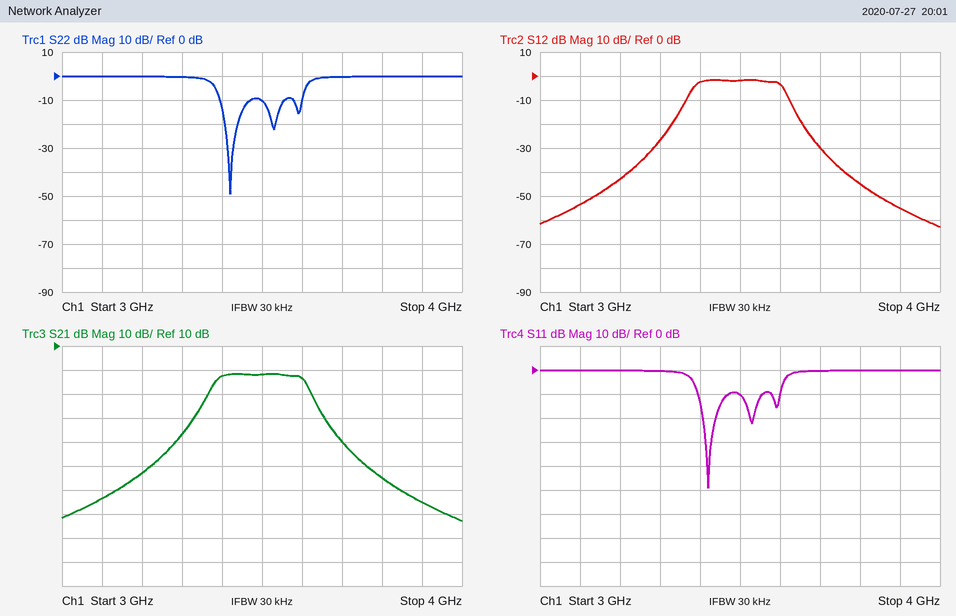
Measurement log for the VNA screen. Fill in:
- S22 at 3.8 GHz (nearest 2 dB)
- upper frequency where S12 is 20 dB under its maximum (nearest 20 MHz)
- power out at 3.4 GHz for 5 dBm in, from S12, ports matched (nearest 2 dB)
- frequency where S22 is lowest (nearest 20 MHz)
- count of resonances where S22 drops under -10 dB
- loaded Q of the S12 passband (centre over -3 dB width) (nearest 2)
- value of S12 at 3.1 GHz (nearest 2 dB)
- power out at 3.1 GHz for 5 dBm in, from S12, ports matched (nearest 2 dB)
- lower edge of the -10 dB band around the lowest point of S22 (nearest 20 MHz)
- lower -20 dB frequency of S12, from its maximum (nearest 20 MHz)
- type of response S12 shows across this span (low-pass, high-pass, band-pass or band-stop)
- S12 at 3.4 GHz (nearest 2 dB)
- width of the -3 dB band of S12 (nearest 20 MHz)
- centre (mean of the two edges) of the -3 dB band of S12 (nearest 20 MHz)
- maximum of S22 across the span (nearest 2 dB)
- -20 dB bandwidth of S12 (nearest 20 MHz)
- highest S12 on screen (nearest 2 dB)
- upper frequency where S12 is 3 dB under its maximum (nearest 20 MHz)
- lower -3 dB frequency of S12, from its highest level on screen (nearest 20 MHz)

0 dB
3.66 GHz
2 dBm
3.42 GHz
3
16
-54 dB
-48 dBm
3.40 GHz
3.32 GHz
band-pass
-2 dB
220 MHz
3.50 GHz
0 dB
340 MHz
-2 dB
3.60 GHz
3.38 GHz
